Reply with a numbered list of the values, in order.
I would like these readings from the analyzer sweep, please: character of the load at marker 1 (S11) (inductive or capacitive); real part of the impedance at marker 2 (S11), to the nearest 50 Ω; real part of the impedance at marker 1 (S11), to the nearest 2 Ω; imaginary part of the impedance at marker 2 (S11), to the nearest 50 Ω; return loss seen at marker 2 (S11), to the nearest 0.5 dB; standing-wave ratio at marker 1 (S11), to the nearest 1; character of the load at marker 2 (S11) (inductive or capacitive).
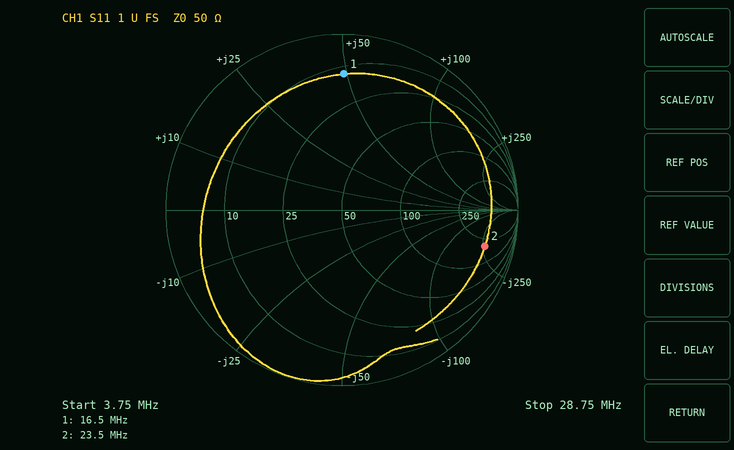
1. inductive
2. 200 Ω
3. 12 Ω
4. -250 Ω
5. 1.5 dB
6. 8
7. capacitive
